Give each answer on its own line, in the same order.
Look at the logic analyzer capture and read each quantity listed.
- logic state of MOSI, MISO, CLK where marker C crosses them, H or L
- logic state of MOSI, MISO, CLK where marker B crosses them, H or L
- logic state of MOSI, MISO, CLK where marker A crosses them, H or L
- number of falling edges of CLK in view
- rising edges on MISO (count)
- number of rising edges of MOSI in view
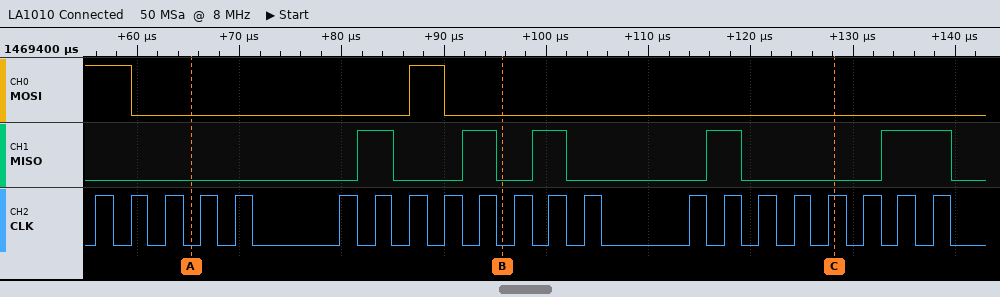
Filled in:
MOSI=L, MISO=L, CLK=H
MOSI=L, MISO=L, CLK=L
MOSI=L, MISO=L, CLK=L
21
5
1
